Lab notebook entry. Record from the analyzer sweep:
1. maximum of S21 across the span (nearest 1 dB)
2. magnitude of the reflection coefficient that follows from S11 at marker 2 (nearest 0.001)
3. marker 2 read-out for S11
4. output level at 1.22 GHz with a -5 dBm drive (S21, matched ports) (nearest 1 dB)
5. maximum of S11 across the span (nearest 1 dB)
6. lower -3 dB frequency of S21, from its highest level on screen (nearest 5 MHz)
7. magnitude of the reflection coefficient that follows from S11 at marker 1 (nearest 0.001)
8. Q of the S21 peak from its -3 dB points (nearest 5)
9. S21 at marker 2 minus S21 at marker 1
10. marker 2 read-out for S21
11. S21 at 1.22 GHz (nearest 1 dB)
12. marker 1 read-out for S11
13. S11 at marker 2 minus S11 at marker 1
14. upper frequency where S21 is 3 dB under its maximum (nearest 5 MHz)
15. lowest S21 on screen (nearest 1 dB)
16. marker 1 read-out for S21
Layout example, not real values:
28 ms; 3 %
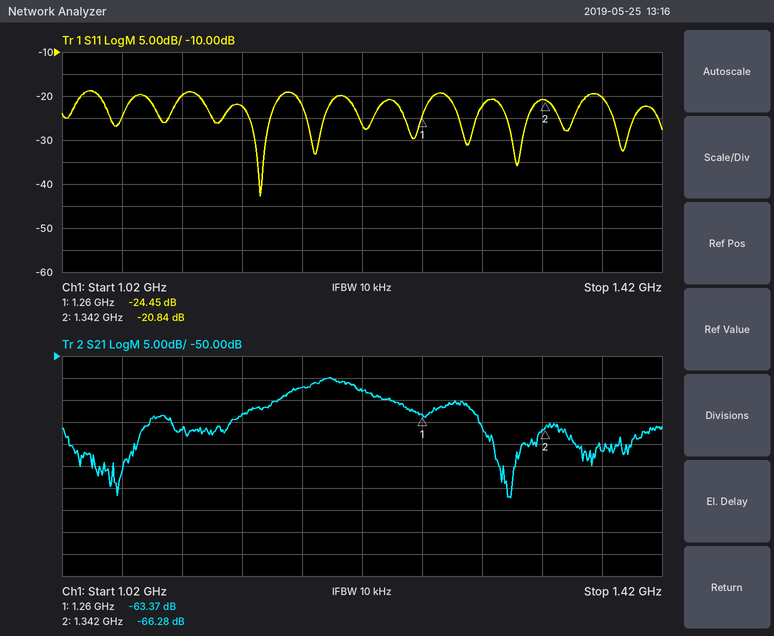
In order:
-55 dB; 0.091; -20.84 dB; -63 dBm; -19 dB; 1.175 GHz; 0.060; 25; -2.91 dB; -66.28 dB; -58 dB; -24.45 dB; 3.61 dB; 1.220 GHz; -82 dB; -63.37 dB
